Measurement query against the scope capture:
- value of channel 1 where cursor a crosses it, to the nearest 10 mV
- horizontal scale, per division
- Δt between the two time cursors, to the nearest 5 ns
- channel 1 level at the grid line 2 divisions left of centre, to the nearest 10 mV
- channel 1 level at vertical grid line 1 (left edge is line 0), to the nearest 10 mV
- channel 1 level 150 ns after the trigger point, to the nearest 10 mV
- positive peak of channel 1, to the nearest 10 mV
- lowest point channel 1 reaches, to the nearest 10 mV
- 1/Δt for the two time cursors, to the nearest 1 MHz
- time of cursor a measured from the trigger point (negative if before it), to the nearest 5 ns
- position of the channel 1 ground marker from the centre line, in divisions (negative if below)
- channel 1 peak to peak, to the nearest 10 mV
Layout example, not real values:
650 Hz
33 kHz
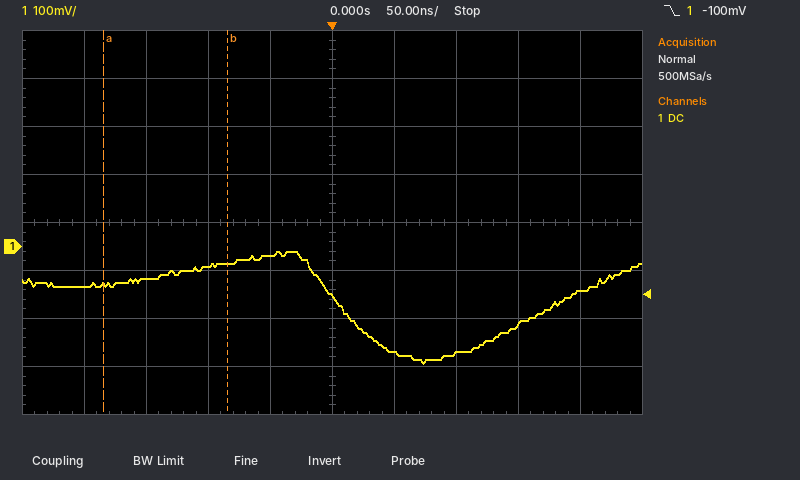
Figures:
-80 mV
50 ns
100 ns
-40 mV
-80 mV
-160 mV
-10 mV
-240 mV
10 MHz
-185 ns
-0.5 div
230 mV
